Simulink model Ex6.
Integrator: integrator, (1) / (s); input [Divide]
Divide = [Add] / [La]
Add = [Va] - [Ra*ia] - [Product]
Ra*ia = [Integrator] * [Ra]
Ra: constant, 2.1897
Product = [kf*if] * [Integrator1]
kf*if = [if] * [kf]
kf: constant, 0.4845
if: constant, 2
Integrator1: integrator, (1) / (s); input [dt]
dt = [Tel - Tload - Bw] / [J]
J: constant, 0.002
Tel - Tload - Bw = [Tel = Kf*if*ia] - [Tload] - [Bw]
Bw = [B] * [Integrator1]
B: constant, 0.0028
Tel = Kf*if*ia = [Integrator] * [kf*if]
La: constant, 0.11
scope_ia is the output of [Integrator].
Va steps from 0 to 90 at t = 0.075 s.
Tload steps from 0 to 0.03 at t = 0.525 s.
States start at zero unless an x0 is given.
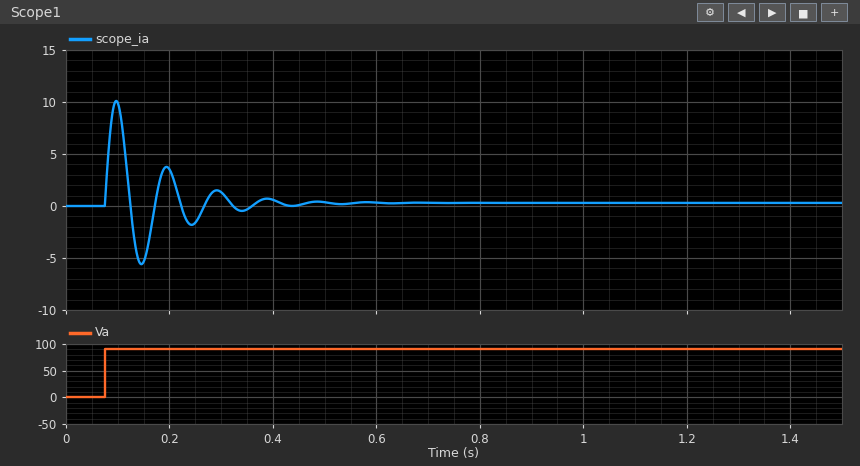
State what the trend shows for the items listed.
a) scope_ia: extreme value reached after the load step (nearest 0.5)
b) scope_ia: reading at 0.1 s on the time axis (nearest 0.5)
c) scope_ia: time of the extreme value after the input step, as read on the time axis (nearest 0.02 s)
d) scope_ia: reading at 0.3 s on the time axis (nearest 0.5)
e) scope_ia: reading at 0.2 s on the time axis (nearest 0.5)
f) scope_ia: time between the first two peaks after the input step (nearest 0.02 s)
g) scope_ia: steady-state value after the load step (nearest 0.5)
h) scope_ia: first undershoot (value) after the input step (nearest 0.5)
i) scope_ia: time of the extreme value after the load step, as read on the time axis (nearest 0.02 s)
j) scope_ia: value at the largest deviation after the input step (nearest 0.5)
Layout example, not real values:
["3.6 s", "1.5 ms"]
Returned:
["0.0", "10.0", "0.10 s", "1.5", "3.5", "0.10 s", "0.5", "-5.5", "0.54 s", "10.0"]
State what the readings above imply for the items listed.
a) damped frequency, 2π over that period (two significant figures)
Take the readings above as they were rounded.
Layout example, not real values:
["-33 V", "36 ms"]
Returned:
["63 rad/s"]
